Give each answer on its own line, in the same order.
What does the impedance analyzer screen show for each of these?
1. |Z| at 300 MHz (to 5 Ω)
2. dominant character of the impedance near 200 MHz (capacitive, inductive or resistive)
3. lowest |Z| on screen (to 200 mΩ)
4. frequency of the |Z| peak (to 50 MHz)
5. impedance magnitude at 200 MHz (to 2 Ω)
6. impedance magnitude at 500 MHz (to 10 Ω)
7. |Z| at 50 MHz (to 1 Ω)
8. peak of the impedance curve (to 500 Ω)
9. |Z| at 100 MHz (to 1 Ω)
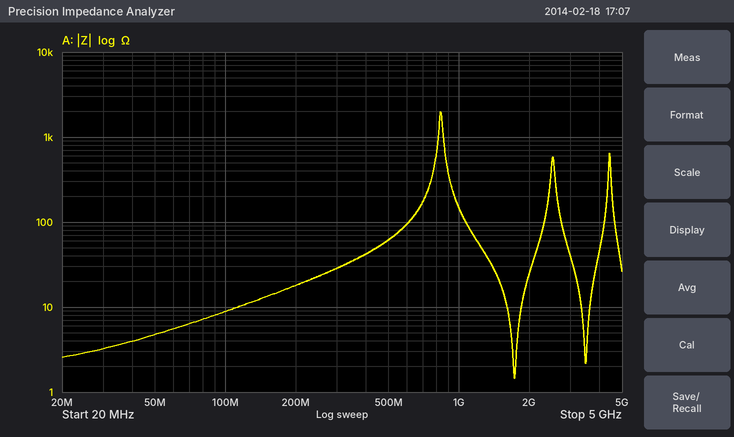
30 Ω
inductive
1.4 Ω
850 MHz
18 Ω
60 Ω
5 Ω
2.0 kΩ
9 Ω
